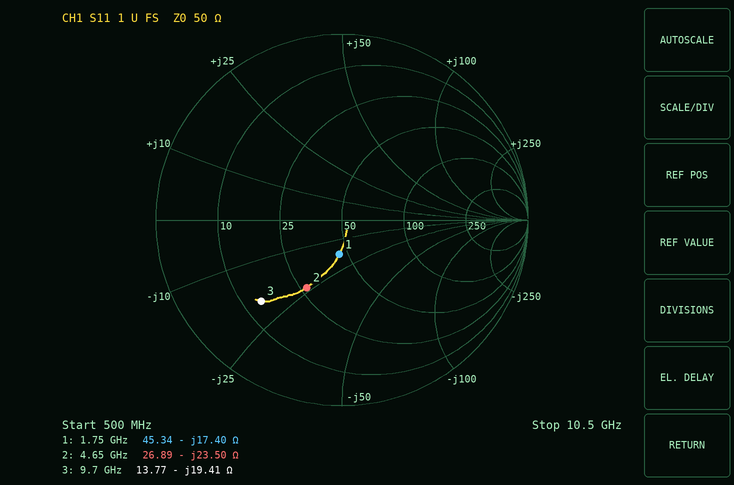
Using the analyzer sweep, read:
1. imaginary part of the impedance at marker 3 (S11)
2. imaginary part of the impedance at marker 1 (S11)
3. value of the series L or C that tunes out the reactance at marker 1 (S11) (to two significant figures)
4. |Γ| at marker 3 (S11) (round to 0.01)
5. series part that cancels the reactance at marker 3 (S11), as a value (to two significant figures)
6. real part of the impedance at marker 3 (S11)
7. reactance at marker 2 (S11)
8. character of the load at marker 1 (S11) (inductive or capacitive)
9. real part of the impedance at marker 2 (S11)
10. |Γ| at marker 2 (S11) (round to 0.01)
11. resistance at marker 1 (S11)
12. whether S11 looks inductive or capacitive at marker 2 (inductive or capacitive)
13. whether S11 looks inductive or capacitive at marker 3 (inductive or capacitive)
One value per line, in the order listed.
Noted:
-19.41 Ω
-17.40 Ω
1.6 nH
0.62
320 pH
13.77 Ω
-23.50 Ω
capacitive
26.89 Ω
0.41
45.34 Ω
capacitive
capacitive
